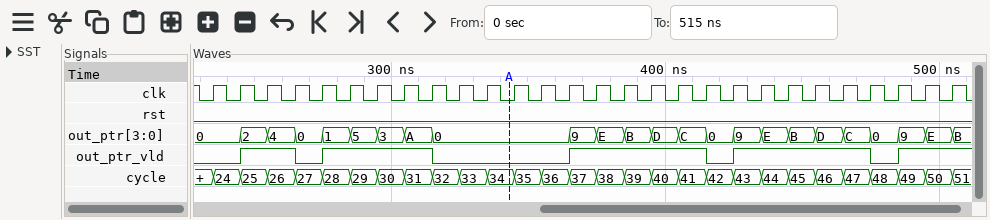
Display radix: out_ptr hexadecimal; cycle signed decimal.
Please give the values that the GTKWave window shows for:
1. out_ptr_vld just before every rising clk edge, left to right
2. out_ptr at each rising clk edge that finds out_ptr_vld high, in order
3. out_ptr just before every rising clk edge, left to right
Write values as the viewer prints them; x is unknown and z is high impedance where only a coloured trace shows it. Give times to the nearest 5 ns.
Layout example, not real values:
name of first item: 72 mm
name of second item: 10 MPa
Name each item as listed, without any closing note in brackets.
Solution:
out_ptr_vld just before every rising clk edge, left to right: 0 0 1 1 0 1 1 1 1 0 0 0 0 0 1 1 1 1 1 0 1 1 1 1 1 0 1 1
out_ptr at each rising clk edge that finds out_ptr_vld high, in order: 2, 4, 1, 5, 3, A, 9, E, B, D, C, 9, E, B, D, C, 9, E
out_ptr just before every rising clk edge, left to right: 0, 0, 2, 4, 0, 1, 5, 3, A, 0, 0, 0, 0, 0, 9, E, B, D, C, 0, 9, E, B, D, C, 0, 9, E
